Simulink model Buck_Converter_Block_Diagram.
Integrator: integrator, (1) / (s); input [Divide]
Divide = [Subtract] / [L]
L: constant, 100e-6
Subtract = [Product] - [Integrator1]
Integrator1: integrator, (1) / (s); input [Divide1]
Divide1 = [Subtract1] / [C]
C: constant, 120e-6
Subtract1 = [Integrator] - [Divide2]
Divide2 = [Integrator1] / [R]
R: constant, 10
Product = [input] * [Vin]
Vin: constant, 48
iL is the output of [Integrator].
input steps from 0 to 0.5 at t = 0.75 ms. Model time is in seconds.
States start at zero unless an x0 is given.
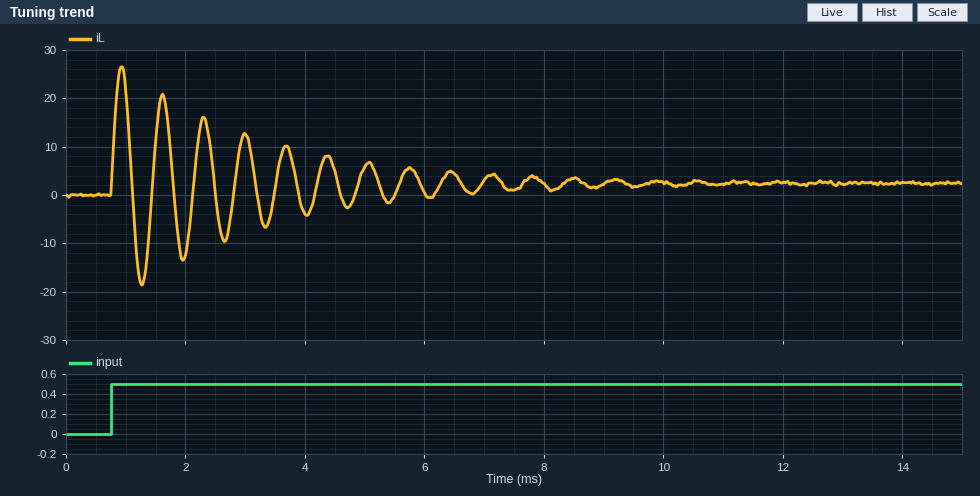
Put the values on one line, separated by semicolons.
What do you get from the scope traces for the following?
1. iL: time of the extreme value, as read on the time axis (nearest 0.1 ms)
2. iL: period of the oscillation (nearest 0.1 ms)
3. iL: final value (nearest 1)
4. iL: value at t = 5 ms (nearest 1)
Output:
0.9 ms; 0.7 ms; 2; 6
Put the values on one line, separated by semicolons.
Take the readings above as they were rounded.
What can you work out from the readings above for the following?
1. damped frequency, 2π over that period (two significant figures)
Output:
9.0 rad/ms
